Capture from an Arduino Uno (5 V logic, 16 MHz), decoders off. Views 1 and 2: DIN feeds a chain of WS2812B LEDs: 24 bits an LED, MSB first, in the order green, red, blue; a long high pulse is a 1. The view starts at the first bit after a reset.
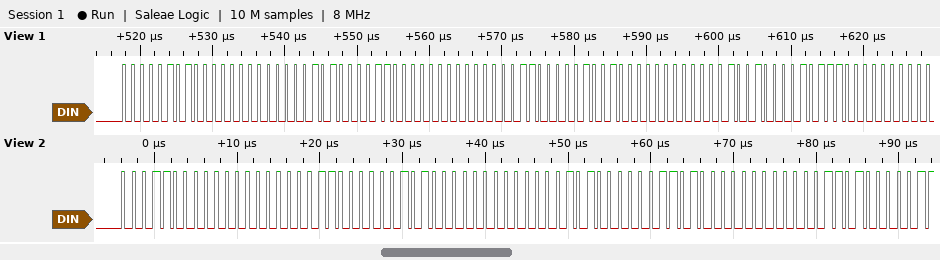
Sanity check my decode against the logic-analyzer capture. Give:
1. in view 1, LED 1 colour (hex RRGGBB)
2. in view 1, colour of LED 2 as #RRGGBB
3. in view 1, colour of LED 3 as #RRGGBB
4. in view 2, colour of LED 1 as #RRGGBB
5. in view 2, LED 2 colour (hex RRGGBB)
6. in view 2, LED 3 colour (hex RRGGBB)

#000505
#000C0C
#001212
#001818
#001414
#000D0D
